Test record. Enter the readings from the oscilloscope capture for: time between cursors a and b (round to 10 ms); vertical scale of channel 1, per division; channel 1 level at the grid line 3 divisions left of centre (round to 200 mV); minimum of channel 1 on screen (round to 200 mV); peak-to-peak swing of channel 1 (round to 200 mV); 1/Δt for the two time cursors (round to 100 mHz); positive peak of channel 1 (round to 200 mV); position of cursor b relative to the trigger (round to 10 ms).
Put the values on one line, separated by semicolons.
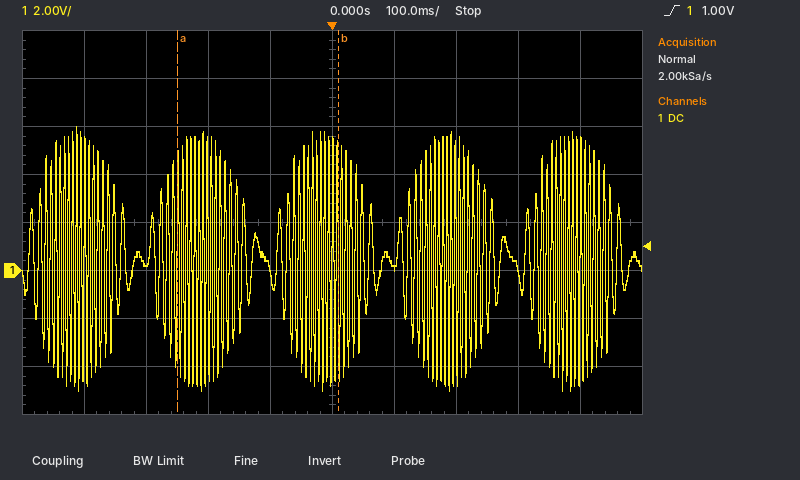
260 ms; 2 V; 400 mV; -5.0 V; 11.0 V; 3.8 Hz; 6.0 V; +10 ms
